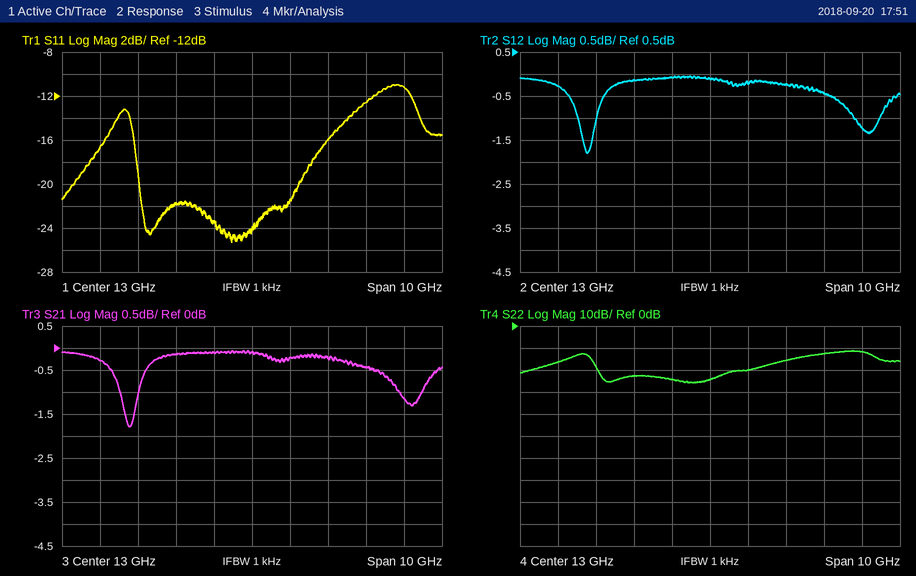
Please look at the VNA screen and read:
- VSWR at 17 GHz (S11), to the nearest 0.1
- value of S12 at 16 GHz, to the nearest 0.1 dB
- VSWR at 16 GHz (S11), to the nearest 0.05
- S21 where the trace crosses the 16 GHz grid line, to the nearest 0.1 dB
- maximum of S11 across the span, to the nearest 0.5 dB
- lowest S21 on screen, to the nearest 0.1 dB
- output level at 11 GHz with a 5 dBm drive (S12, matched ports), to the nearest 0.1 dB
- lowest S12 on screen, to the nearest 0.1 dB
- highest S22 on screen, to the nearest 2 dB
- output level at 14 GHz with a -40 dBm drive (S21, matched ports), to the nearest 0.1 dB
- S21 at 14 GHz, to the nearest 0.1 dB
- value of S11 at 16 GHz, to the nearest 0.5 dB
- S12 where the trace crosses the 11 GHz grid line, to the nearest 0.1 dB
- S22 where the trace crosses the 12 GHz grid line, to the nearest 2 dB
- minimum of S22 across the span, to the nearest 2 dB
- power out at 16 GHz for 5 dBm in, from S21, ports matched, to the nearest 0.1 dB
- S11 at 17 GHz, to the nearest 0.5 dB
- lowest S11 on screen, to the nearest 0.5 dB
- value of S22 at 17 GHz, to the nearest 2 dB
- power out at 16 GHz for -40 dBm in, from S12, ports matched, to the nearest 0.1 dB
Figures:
1.8
-0.4 dB
1.60
-0.4 dB
-11.0 dB
-1.8 dB
4.9 dBm
-1.8 dB
-12 dB
-40.2 dBm
-0.2 dB
-12.5 dB
-0.1 dB
-24 dB
-26 dB
4.6 dBm
-11.0 dB
-25.5 dB
-12 dB
-40.4 dBm
